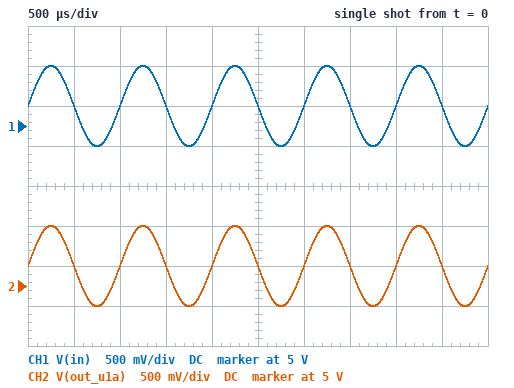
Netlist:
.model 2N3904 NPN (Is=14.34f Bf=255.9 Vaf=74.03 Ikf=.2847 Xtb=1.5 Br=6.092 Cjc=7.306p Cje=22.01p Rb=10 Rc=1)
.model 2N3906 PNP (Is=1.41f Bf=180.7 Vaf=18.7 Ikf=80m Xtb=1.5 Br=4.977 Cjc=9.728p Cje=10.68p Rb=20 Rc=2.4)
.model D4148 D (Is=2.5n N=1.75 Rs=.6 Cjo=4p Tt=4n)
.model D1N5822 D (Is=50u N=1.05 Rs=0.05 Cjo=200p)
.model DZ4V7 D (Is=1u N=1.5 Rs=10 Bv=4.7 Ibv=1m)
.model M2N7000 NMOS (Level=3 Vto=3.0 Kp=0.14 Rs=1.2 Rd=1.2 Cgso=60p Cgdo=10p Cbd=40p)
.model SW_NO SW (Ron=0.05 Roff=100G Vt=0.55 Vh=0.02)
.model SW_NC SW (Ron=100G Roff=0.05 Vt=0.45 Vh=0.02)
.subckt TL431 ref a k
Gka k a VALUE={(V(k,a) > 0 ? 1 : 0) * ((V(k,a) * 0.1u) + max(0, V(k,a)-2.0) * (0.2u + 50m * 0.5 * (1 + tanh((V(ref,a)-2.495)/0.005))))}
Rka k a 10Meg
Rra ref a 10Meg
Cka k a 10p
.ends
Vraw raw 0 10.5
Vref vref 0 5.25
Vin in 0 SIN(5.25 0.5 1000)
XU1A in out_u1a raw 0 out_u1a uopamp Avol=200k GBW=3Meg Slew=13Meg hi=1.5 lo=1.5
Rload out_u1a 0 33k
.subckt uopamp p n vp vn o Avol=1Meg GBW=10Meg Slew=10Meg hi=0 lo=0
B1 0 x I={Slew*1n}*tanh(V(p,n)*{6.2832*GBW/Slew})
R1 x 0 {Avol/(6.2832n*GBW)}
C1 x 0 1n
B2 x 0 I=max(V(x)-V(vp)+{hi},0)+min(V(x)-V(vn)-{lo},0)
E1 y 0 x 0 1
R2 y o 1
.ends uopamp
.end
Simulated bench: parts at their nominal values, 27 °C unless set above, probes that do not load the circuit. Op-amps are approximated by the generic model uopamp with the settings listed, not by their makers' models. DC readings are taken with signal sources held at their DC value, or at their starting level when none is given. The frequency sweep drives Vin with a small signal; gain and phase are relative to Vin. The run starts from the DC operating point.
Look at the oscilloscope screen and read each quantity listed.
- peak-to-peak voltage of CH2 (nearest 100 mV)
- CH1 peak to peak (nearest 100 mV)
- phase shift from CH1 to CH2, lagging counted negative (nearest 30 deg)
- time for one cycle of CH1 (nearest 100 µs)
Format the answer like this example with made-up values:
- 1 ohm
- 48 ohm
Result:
- 1.0 V
- 1.0 V
- 0 deg
- 1.0 ms
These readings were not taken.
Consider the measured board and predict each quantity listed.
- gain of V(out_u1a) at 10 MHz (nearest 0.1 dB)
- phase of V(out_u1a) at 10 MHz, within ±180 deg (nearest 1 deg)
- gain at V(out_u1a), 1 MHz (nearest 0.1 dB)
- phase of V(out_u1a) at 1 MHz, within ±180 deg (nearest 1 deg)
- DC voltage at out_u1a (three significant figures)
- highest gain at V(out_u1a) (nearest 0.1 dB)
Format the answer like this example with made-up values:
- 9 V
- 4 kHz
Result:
- -10.8 dB
- -73 deg
- -0.5 dB
- -18 deg
- 5.25 V
- 0 dB
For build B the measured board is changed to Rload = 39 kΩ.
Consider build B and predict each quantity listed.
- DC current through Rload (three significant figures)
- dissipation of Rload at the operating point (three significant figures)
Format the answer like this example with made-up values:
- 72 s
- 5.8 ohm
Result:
- 135 µA
- 707 µW
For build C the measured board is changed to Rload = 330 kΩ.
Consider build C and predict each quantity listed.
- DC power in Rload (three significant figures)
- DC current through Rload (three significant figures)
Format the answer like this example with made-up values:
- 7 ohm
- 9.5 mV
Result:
- 83.5 µW
- 15.9 µA
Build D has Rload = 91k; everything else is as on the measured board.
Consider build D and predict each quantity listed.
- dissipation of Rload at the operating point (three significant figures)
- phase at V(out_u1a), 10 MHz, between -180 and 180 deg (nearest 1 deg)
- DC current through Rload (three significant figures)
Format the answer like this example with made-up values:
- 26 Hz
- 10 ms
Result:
- 303 µW
- -73 deg
- 57.7 µA
